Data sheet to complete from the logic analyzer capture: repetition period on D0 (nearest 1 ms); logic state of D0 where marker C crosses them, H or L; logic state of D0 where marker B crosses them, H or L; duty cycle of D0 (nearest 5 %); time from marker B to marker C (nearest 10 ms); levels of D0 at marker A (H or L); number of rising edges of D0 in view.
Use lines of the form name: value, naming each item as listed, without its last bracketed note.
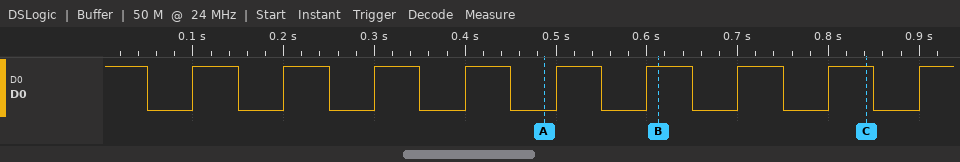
repetition period on D0: 100 ms
logic state of D0 where marker C crosses them, H or L: D0=H
logic state of D0 where marker B crosses them, H or L: D0=H
duty cycle of D0: 50 %
time from marker B to marker C: 230 ms
levels of D0 at marker A: D0=L
number of rising edges of D0 in view: 9
